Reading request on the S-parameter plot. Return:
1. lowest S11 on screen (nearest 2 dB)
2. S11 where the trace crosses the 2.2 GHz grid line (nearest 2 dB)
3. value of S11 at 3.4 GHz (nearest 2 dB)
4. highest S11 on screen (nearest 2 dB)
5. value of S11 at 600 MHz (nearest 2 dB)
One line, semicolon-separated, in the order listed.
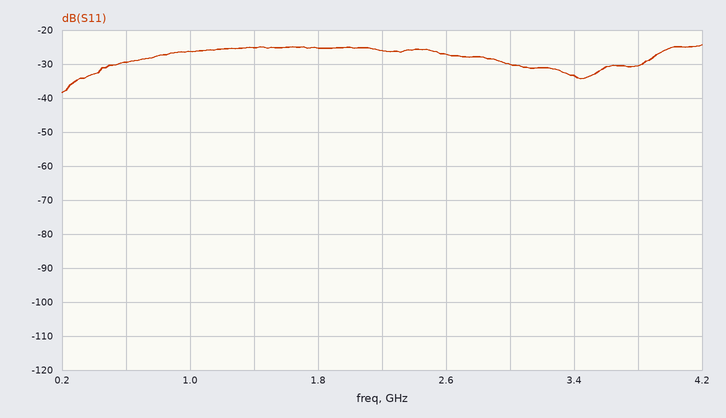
-38 dB; -26 dB; -34 dB; -24 dB; -30 dB
